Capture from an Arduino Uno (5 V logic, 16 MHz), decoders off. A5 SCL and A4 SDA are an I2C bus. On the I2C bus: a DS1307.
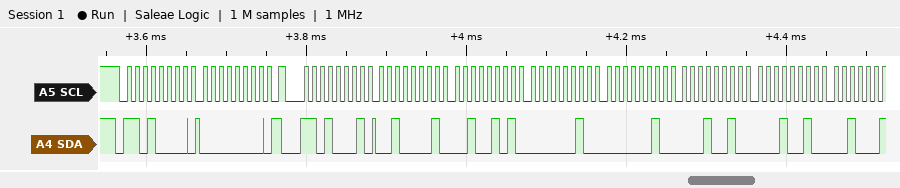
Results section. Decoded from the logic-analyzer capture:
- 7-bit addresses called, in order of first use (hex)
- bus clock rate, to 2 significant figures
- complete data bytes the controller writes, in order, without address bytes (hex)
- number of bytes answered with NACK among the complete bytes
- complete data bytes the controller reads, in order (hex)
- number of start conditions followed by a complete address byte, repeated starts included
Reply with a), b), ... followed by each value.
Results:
a) 0x68
b) 100 kHz
c) 00
d) 0
e) 21 25 02 02 12 12
f) 2
